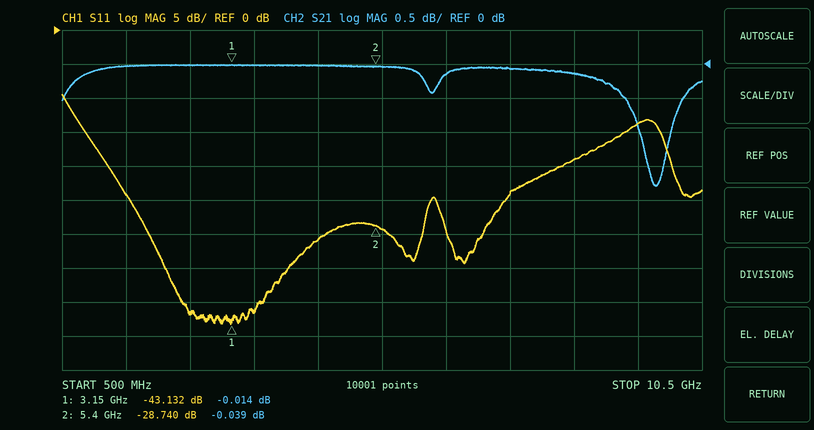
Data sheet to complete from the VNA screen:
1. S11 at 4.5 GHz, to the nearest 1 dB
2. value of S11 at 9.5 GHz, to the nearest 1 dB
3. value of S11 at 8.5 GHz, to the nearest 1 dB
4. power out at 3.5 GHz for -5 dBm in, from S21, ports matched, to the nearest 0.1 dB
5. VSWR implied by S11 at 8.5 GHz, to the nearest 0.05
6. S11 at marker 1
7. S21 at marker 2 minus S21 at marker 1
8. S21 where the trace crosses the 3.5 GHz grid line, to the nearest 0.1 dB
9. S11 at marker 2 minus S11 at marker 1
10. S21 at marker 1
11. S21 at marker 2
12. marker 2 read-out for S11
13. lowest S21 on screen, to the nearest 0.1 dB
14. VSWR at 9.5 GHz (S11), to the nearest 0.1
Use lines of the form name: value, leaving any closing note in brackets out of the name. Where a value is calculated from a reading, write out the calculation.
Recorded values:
S11 at 4.5 GHz, to the nearest 1 dB: -31 dB
value of S11 at 9.5 GHz, to the nearest 1 dB: -14 dB
value of S11 at 8.5 GHz, to the nearest 1 dB: -19 dB
power out at 3.5 GHz for -5 dBm in, from S21, ports matched, to the nearest 0.1 dB: -5 dBm + (0.0 dB) = -5.0 dBm
VSWR implied by S11 at 8.5 GHz, to the nearest 0.05: |Γ| = 10^(-19/20) = 0.1122; VSWR = (1 + 0.1122)/(1 − 0.1122) ≈ 1.25
S11 at marker 1: -43.132 dB
S21 at marker 2 minus S21 at marker 1: -0.039 − (-0.014) = -0.025 dB
S21 where the trace crosses the 3.5 GHz grid line, to the nearest 0.1 dB: 0.0 dB
S11 at marker 2 minus S11 at marker 1: -28.74 − (-43.132) = 14.392 dB
S21 at marker 1: -0.014 dB
S21 at marker 2: -0.039 dB
marker 2 read-out for S11: -28.740 dB
lowest S21 on screen, to the nearest 0.1 dB: -1.8 dB
VSWR at 9.5 GHz (S11), to the nearest 0.1: |Γ| = 10^(-14/20) = 0.1995; VSWR = (1 + 0.1995)/(1 − 0.1995) ≈ 1.5
